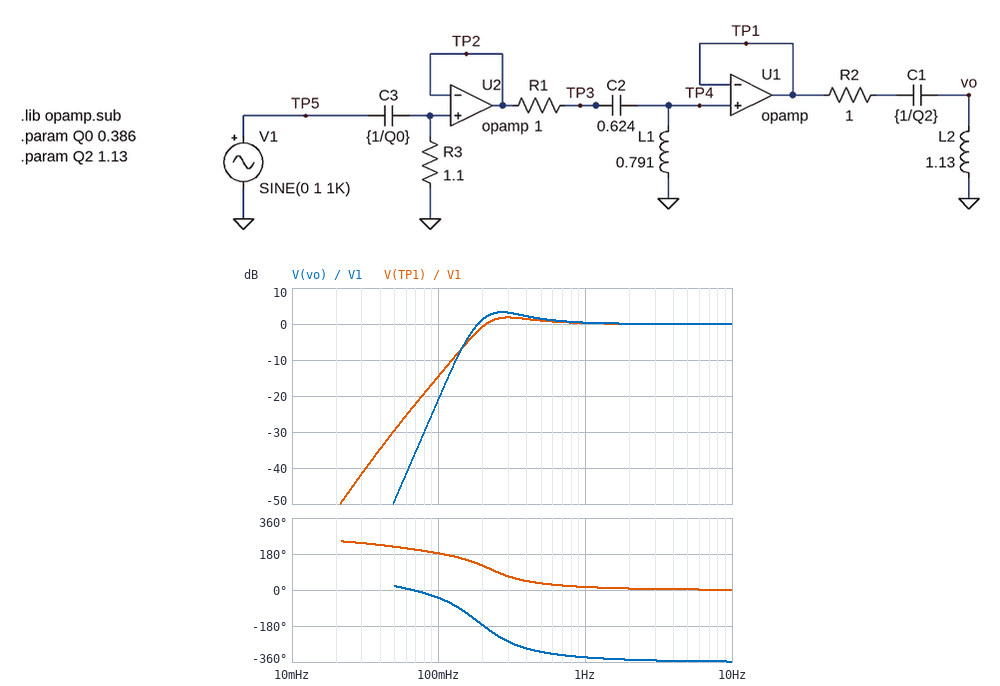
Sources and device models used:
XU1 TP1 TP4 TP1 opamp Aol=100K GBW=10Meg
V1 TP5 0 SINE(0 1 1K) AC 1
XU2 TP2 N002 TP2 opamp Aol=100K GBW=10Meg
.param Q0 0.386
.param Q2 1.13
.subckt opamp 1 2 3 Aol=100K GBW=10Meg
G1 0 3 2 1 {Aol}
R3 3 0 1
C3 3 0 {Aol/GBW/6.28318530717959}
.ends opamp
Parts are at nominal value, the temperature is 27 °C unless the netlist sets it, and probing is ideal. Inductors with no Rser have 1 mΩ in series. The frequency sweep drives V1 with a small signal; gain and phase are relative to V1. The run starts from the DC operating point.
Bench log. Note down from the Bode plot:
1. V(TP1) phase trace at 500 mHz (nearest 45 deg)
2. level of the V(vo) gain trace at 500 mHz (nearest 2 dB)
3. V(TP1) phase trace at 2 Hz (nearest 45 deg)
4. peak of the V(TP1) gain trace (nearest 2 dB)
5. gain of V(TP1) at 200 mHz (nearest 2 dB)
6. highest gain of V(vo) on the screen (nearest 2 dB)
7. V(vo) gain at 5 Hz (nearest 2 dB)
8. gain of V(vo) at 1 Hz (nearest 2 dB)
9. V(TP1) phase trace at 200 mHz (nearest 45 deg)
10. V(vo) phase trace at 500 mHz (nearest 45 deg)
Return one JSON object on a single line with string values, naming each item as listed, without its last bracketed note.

{"V(TP1) phase trace at 500 mHz": "45 deg", "level of the V(vo) gain trace at 500 mHz": "2 dB", "V(TP1) phase trace at 2 Hz": "0 deg", "peak of the V(TP1) gain trace": "2 dB", "gain of V(TP1) at 200 mHz": "0 dB", "highest gain of V(vo) on the screen": "4 dB", "V(vo) gain at 5 Hz": "0 dB", "gain of V(vo) at 1 Hz": "0 dB", "V(TP1) phase trace at 200 mHz": "135 deg", "V(vo) phase trace at 500 mHz": "-315 deg"}
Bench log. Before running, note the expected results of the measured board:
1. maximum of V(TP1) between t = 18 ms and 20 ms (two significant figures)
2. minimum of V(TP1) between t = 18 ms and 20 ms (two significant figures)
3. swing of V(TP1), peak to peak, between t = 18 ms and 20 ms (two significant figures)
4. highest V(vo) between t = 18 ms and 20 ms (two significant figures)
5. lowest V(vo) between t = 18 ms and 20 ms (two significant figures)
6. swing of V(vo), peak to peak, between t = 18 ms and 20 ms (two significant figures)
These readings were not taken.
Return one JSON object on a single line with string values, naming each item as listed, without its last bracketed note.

{"maximum of V(TP1) between t = 18 ms and 20 ms": "1.0 V", "minimum of V(TP1) between t = 18 ms and 20 ms": "-1.0 V", "swing of V(TP1), peak to peak, between t = 18 ms and 20 ms": "2.0 V", "highest V(vo) between t = 18 ms and 20 ms": "1.0 V", "lowest V(vo) between t = 18 ms and 20 ms": "-1.0 V", "swing of V(vo), peak to peak, between t = 18 ms and 20 ms": "2.0 V"}
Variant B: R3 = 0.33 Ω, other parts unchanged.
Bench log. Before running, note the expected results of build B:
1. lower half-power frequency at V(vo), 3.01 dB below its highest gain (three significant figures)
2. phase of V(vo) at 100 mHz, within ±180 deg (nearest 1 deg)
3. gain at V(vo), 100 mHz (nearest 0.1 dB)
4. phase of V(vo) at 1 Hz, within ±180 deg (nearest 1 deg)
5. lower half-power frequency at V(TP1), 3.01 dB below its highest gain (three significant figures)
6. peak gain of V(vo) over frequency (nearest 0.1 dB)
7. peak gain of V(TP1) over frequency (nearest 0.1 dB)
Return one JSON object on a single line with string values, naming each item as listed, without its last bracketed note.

{"lower half-power frequency at V(vo), 3.01 dB below its highest gain": "200 mHz", "phase of V(vo) at 100 mHz, within ±180 deg": "-7 deg", "gain at V(vo), 100 mHz": "-26.1 dB", "phase of V(vo) at 1 Hz, within ±180 deg": "31 deg", "lower half-power frequency at V(TP1), 3.01 dB below its highest gain": "209 mHz", "peak gain of V(vo) over frequency": "1.9 dB", "peak gain of V(TP1) over frequency": "0.7 dB"}
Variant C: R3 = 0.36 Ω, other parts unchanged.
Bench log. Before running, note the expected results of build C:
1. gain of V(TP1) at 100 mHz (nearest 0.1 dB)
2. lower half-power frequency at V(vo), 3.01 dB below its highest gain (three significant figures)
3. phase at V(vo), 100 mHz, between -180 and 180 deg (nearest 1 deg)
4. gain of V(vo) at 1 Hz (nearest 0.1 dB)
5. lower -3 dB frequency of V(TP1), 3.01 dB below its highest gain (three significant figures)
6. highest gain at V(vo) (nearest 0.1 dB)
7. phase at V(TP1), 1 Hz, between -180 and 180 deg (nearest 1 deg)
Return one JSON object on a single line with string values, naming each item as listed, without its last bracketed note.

{"gain of V(TP1) at 100 mHz": "-19.2 dB", "lower half-power frequency at V(vo), 3.01 dB below its highest gain": "198 mHz", "phase at V(vo), 100 mHz, between -180 and 180 deg": "-9 deg", "gain of V(vo) at 1 Hz": "0.3 dB", "lower -3 dB frequency of V(TP1), 3.01 dB below its highest gain": "207 mHz", "highest gain at V(vo)": "2.1 dB", "phase at V(TP1), 1 Hz, between -180 and 180 deg": "22 deg"}
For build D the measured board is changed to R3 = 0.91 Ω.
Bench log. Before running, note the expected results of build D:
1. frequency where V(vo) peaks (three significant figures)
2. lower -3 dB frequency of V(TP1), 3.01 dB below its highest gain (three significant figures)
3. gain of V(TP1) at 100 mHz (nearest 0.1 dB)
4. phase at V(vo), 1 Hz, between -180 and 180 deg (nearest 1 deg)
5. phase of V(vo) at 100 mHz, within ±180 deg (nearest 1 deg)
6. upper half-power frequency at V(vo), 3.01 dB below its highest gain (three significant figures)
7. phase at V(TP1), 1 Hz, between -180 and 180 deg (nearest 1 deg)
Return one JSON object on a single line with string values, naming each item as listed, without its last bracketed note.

{"frequency where V(vo) peaks": "271 mHz", "lower -3 dB frequency of V(TP1), 3.01 dB below its highest gain": "195 mHz", "gain of V(TP1) at 100 mHz": "-14.9 dB", "phase at V(vo), 1 Hz, between -180 and 180 deg": "24 deg", "phase of V(vo) at 100 mHz, within ±180 deg": "-35 deg", "upper half-power frequency at V(vo), 3.01 dB below its highest gain": "1.40 Hz", "phase at V(TP1), 1 Hz, between -180 and 180 deg": "16 deg"}
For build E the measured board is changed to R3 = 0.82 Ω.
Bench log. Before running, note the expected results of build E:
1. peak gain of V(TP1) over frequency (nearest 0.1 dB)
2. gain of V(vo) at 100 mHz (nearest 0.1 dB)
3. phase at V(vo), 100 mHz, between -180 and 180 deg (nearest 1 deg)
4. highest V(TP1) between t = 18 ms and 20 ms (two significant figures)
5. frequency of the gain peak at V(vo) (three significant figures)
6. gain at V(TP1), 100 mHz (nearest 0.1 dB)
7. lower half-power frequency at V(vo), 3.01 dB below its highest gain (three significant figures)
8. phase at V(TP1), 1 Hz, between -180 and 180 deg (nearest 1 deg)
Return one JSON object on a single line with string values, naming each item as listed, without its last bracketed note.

{"peak gain of V(TP1) over frequency": "1.7 dB", "gain of V(vo) at 100 mHz": "-21.6 dB", "phase at V(vo), 100 mHz, between -180 and 180 deg": "-32 deg", "highest V(TP1) between t = 18 ms and 20 ms": "1.0 V", "frequency of the gain peak at V(vo)": "272 mHz", "gain at V(TP1), 100 mHz": "-15.2 dB", "lower half-power frequency at V(vo), 3.01 dB below its highest gain": "190 mHz", "phase at V(TP1), 1 Hz, between -180 and 180 deg": "16 deg"}
